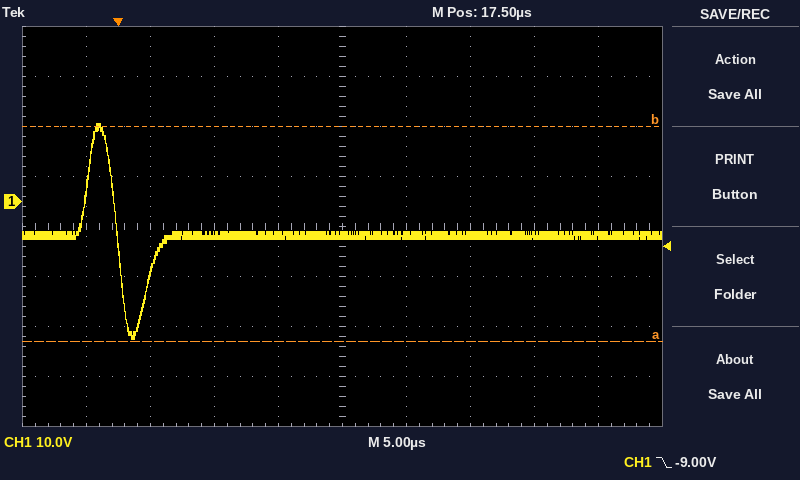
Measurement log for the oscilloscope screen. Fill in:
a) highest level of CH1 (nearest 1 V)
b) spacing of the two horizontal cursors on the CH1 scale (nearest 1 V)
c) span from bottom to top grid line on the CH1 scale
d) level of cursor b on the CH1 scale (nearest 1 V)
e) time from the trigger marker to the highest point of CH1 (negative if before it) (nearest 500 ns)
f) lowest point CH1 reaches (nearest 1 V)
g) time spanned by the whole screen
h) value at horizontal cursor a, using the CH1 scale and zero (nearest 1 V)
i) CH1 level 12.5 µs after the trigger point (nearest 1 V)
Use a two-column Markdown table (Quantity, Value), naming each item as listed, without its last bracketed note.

| Quantity | Value |
|---|---|
| highest level of CH1 | 16 V |
| spacing of the two horizontal cursors on the CH1 scale | 43 V |
| span from bottom to top grid line on the CH1 scale | 80 V |
| level of cursor b on the CH1 scale | 15 V |
| time from the trigger marker to the highest point of CH1 (negative if before it) | -1.5 µs |
| lowest point CH1 reaches | -28 V |
| time spanned by the whole screen | 50 µs |
| value at horizontal cursor a, using the CH1 scale and zero | -28 V |
| CH1 level 12.5 µs after the trigger point | -7 V |
